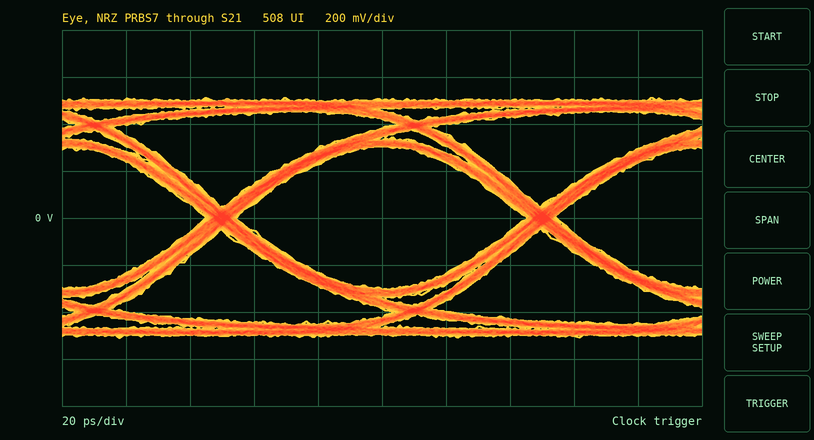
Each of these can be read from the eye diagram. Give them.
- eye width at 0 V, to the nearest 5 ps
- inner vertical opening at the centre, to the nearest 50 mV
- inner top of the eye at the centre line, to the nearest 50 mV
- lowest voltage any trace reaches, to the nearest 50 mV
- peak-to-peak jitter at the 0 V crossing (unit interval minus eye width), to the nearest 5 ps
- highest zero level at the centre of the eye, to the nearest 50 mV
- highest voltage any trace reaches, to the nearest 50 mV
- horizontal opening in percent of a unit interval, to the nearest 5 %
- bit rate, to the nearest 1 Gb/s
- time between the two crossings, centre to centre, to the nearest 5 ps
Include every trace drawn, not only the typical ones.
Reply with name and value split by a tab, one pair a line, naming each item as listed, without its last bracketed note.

eye width at 0 V, to the nearest 5 ps	90 ps
inner vertical opening at the centre, to the nearest 50 mV	600 mV
inner top of the eye at the centre line, to the nearest 50 mV	300 mV
lowest voltage any trace reaches, to the nearest 50 mV	-500 mV
peak-to-peak jitter at the 0 V crossing (unit interval minus eye width), to the nearest 5 ps	10 ps
highest zero level at the centre of the eye, to the nearest 50 mV	-300 mV
highest voltage any trace reaches, to the nearest 50 mV	500 mV
horizontal opening in percent of a unit interval, to the nearest 5 %	90 %
bit rate, to the nearest 1 Gb/s	10 Gb/s
time between the two crossings, centre to centre, to the nearest 5 ps	100 ps
